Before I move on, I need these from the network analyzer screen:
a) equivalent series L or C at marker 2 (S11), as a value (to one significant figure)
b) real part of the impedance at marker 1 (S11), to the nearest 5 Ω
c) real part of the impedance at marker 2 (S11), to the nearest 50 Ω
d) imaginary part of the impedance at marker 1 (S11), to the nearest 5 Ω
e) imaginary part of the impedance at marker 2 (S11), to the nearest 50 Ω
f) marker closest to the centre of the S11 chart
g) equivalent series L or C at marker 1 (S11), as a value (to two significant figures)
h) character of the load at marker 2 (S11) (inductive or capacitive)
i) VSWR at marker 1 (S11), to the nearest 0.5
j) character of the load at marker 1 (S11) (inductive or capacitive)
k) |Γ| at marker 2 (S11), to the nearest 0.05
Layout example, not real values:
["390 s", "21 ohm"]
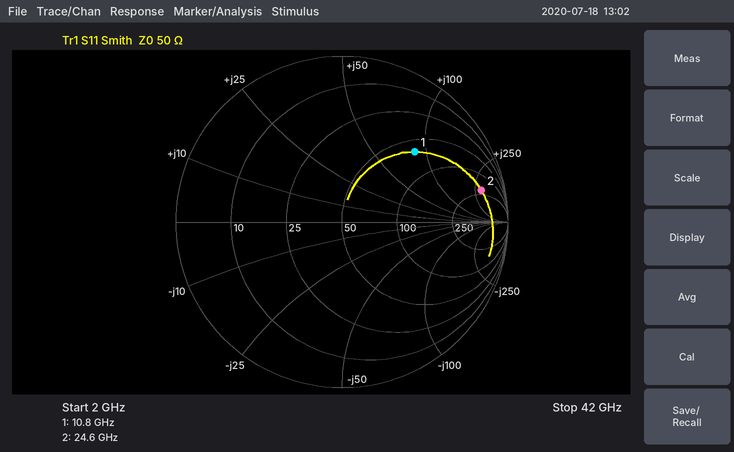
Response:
["2 nH", "65 Ω", "200 Ω", "+85 Ω", "+300 Ω", "marker 1", "1.3 nH", "inductive", "4.0", "inductive", "0.85"]
